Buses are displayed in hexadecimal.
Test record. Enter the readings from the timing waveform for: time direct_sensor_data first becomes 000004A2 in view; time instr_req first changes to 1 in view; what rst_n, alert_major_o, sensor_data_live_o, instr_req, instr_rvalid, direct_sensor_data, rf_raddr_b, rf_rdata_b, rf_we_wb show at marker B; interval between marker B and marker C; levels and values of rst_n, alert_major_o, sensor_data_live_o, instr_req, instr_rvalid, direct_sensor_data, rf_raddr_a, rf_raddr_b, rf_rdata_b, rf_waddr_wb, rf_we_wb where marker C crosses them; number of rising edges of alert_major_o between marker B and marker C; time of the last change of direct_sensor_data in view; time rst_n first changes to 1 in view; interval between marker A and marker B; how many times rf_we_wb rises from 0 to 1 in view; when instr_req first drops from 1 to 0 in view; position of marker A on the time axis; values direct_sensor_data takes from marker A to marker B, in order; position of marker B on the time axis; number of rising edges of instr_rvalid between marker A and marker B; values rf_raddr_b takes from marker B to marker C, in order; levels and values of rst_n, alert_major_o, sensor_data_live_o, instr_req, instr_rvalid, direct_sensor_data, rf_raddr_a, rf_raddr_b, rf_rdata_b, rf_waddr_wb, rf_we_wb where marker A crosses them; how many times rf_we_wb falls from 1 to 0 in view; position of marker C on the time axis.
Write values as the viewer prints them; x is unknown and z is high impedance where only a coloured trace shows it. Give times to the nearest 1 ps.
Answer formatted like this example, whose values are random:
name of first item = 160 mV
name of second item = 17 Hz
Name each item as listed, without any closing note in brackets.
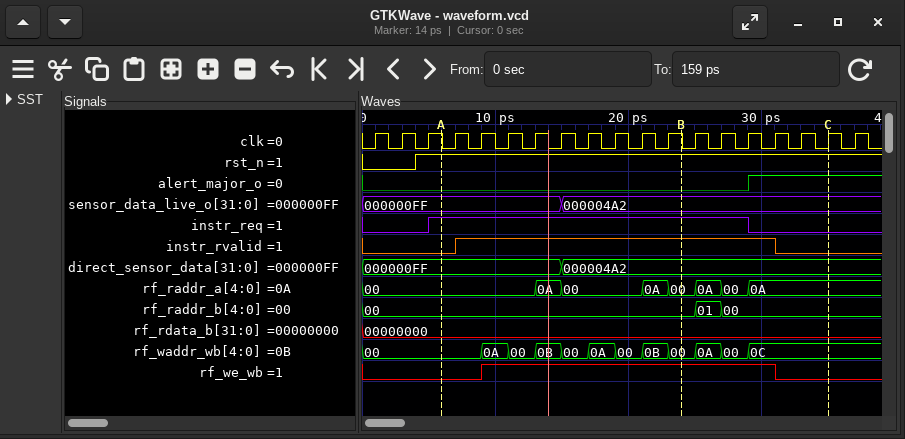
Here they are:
time direct_sensor_data first becomes 000004A2 in view = 15 ps
time instr_req first changes to 1 in view = 5 ps
what rst_n, alert_major_o, sensor_data_live_o, instr_req, instr_rvalid, direct_sensor_data, rf_raddr_b, rf_rdata_b, rf_we_wb show at marker B = rst_n=1, alert_major_o=0, sensor_data_live_o=000004A2, instr_req=1, instr_rvalid=1, direct_sensor_data=000004A2, rf_raddr_b=00, rf_rdata_b=00000000, rf_we_wb=1
interval between marker B and marker C = 11 ps
levels and values of rst_n, alert_major_o, sensor_data_live_o, instr_req, instr_rvalid, direct_sensor_data, rf_raddr_a, rf_raddr_b, rf_rdata_b, rf_waddr_wb, rf_we_wb where marker C crosses them = rst_n=1, alert_major_o=1, sensor_data_live_o=000004A2, instr_req=0, instr_rvalid=0, direct_sensor_data=000004A2, rf_raddr_a=0A, rf_raddr_b=00, rf_rdata_b=00000000, rf_waddr_wb=0C, rf_we_wb=0
number of rising edges of alert_major_o between marker B and marker C = 1
time of the last change of direct_sensor_data in view = 15 ps
time rst_n first changes to 1 in view = 4 ps
interval between marker A and marker B = 18 ps
how many times rf_we_wb rises from 0 to 1 in view = 1
when instr_req first drops from 1 to 0 in view = 29 ps
position of marker A on the time axis = 6 ps
values direct_sensor_data takes from marker A to marker B, in order = 000000FF, 000004A2
position of marker B on the time axis = 24 ps
number of rising edges of instr_rvalid between marker A and marker B = 1
values rf_raddr_b takes from marker B to marker C, in order = 00, 01, 00
levels and values of rst_n, alert_major_o, sensor_data_live_o, instr_req, instr_rvalid, direct_sensor_data, rf_raddr_a, rf_raddr_b, rf_rdata_b, rf_waddr_wb, rf_we_wb where marker A crosses them = rst_n=1, alert_major_o=0, sensor_data_live_o=000000FF, instr_req=1, instr_rvalid=0, direct_sensor_data=000000FF, rf_raddr_a=00, rf_raddr_b=00, rf_rdata_b=00000000, rf_waddr_wb=00, rf_we_wb=0
how many times rf_we_wb falls from 1 to 0 in view = 1
position of marker C on the time axis = 35 ps
